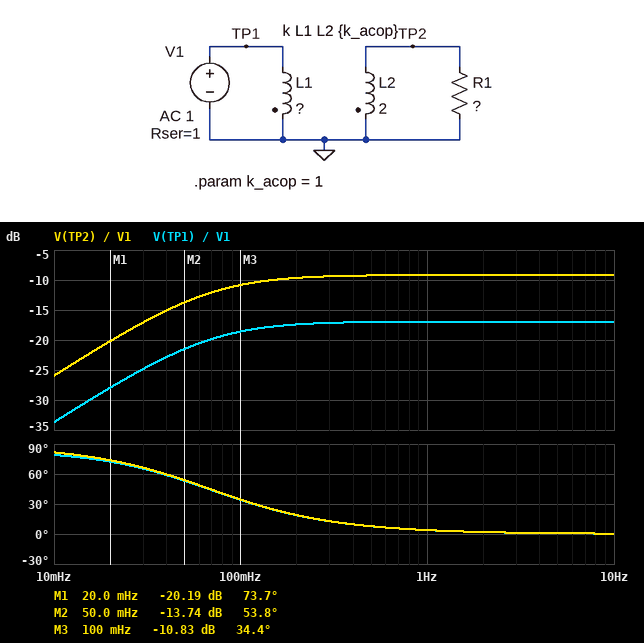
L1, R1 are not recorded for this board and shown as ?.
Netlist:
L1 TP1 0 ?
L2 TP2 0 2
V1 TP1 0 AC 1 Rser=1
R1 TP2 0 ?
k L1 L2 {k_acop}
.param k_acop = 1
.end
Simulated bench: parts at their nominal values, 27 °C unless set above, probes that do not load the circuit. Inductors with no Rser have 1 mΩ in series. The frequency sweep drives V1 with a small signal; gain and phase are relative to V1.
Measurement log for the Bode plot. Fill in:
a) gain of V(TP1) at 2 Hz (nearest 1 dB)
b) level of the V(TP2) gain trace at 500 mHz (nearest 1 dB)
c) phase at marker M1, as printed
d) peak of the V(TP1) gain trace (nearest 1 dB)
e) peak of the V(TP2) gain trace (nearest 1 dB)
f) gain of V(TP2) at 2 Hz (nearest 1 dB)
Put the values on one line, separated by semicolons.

-17 dB; -9 dB; 73.7 deg; -17 dB; -9 dB; -9 dB
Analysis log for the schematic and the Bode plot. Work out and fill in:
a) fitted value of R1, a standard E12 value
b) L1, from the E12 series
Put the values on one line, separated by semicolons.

1 Ω; 330 mH
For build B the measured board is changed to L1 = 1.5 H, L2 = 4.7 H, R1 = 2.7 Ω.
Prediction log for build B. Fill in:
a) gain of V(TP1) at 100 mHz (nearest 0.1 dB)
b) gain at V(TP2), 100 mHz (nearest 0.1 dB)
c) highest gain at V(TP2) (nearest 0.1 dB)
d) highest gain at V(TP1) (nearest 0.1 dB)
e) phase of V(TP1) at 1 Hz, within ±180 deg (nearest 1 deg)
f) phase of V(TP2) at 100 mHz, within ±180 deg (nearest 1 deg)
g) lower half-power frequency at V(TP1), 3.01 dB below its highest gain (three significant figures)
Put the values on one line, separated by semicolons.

-7.6 dB; -2.7 dB; -1.7 dB; -6.7 dB; 3 deg; 26 deg; 49.1 mHz
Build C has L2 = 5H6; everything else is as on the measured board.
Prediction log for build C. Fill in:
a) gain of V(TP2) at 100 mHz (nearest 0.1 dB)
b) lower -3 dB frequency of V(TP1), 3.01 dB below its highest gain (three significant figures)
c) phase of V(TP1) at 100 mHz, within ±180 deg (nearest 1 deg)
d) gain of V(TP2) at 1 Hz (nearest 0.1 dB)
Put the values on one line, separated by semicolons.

-13.1 dB; 26.9 mHz; 15 deg; -12.8 dB
